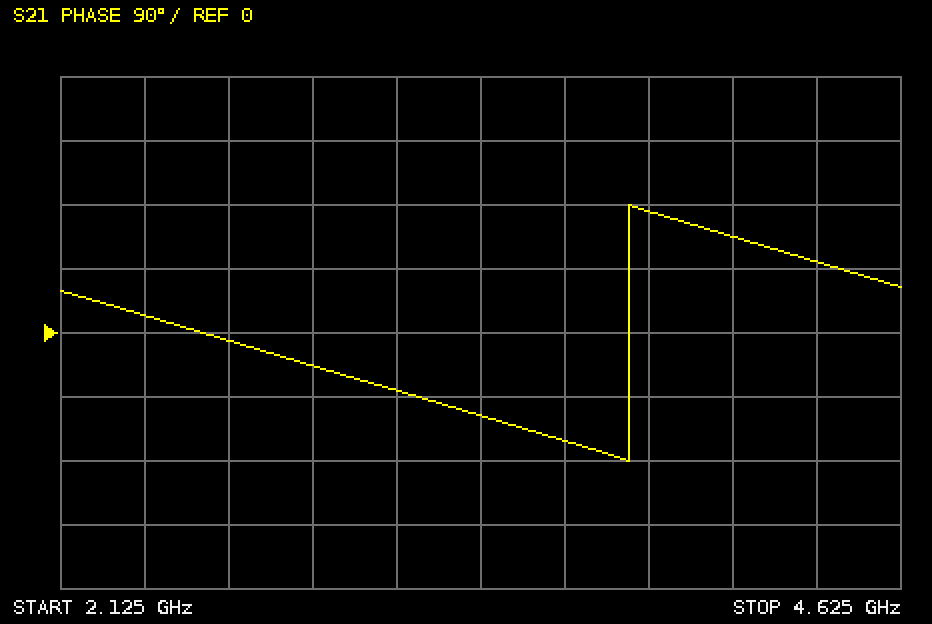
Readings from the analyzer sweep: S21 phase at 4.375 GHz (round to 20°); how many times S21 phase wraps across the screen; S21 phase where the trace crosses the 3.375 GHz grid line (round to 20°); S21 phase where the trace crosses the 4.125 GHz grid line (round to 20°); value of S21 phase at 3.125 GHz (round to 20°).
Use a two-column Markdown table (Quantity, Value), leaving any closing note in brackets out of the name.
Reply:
| Quantity | Value |
|---|---|
| S21 phase at 4.375 GHz | 100° |
| how many times S21 phase wraps across the screen | 1 |
| S21 phase where the trace crosses the 3.375 GHz grid line | -120° |
| S21 phase where the trace crosses the 4.125 GHz grid line | 140° |
| value of S21 phase at 3.125 GHz | -80° |
